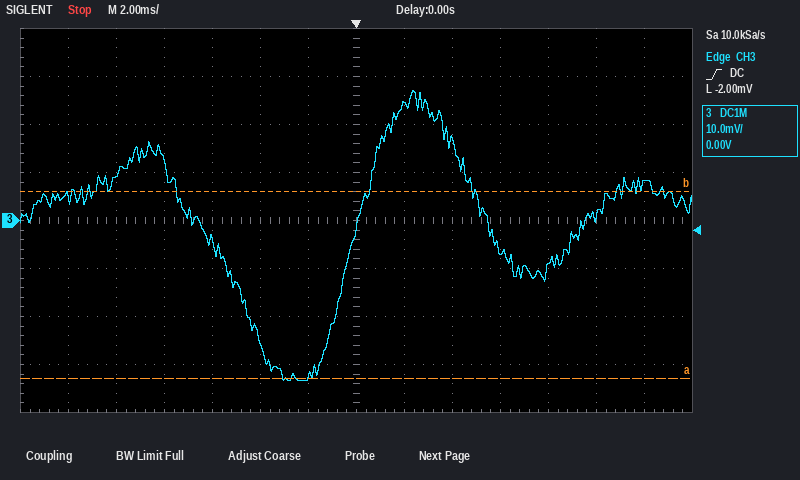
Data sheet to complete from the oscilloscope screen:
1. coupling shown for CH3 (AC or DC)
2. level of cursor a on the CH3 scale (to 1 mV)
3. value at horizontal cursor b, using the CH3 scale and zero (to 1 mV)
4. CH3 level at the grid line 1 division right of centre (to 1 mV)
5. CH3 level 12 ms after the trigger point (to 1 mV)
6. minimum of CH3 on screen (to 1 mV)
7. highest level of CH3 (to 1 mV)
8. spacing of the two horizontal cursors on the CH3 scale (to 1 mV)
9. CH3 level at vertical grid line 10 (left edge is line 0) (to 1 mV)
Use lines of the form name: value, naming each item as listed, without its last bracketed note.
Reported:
coupling shown for CH3: DC
level of cursor a on the CH3 scale: -33 mV
value at horizontal cursor b, using the CH3 scale and zero: 6 mV
CH3 level at the grid line 1 division right of centre: 24 mV
CH3 level 12 ms after the trigger point: 8 mV
minimum of CH3 on screen: -33 mV
highest level of CH3: 27 mV
spacing of the two horizontal cursors on the CH3 scale: 39 mV
CH3 level at vertical grid line 10 (left edge is line 0): -6 mV
